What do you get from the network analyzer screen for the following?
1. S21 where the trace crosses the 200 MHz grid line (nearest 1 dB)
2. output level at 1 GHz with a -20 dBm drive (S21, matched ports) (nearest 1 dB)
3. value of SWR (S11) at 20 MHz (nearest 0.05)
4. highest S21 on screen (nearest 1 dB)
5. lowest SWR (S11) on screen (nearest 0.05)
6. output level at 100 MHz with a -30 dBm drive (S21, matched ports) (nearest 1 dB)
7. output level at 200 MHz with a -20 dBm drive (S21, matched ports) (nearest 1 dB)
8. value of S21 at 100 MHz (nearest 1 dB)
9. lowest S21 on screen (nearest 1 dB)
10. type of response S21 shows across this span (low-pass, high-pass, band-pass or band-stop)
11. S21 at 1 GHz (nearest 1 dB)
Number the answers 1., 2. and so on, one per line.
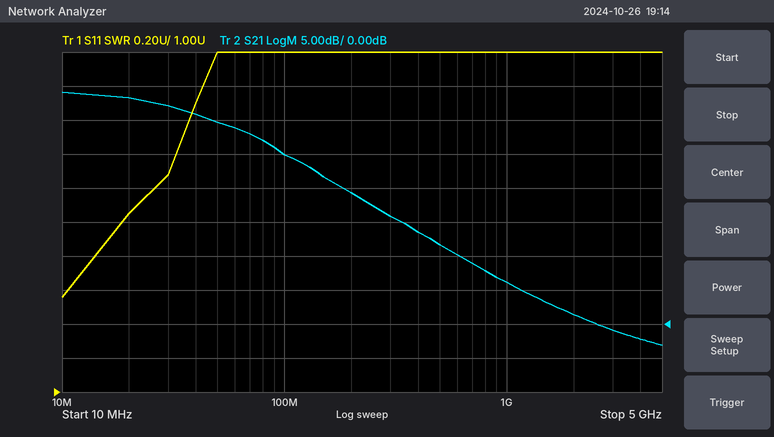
1. 19 dB
2. -14 dBm
3. 2.05
4. 34 dB
5. 1.55
6. -5 dBm
7. -1 dBm
8. 25 dB
9. -3 dB
10. low-pass
11. 6 dB
